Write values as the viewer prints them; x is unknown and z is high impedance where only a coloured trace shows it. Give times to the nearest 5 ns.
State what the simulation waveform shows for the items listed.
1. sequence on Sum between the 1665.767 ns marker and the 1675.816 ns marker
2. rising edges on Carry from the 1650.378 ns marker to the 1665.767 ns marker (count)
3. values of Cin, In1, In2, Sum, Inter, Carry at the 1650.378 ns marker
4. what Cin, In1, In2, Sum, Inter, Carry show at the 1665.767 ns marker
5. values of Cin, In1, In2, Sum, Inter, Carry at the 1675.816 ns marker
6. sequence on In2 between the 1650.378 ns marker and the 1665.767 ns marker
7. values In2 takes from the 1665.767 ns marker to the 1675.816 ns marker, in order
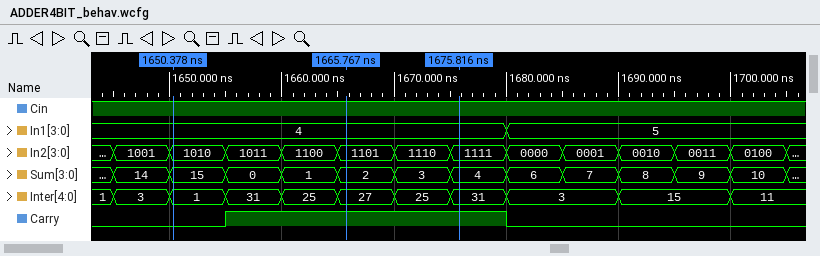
2, 3, 4
1
Cin=1, In1=4, In2=1010, Sum=15, Inter=1, Carry=0
Cin=1, In1=4, In2=1101, Sum=2, Inter=27, Carry=1
Cin=1, In1=4, In2=1111, Sum=4, Inter=31, Carry=1
1010, 1011, 1100, 1101
1101, 1110, 1111
